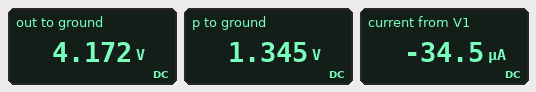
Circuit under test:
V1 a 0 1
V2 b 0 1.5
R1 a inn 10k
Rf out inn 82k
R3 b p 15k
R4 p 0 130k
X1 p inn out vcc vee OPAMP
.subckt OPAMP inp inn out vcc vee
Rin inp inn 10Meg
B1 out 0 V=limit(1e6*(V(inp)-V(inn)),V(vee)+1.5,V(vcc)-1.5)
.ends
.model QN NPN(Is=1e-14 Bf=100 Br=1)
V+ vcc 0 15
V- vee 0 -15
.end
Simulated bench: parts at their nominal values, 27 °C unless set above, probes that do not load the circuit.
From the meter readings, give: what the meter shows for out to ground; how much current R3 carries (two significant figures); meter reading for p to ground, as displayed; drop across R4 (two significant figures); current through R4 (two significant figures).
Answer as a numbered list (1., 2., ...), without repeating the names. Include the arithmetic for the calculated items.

1. 4.172 V
2. (1.5 V - 1.345 V) / 15 kΩ = 10 µA
3. 1.345 V
4. 1.345 V = 1.3 V
5. (1.345 V) / 130 kΩ = 10 µA
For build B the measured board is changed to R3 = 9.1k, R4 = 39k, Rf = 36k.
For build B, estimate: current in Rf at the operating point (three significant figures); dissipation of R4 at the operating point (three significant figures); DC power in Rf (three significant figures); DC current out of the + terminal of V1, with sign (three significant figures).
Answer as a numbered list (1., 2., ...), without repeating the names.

1. 21.6 µA
2. 37.9 µW
3. 16.8 µW
4. -21.6 µA
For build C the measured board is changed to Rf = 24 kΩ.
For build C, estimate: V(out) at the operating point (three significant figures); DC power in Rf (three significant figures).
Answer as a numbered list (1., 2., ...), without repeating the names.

1. 2.17 V
2. 28.5 µW
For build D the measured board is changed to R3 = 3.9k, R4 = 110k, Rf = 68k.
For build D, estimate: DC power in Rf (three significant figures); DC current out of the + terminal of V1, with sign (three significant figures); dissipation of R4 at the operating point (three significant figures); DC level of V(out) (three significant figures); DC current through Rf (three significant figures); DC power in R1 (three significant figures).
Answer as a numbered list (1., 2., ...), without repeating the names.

1. 137 µW
2. -44.9 µA
3. 19.1 µW
4. 4.50 V
5. 44.9 µA
6. 20.1 µW
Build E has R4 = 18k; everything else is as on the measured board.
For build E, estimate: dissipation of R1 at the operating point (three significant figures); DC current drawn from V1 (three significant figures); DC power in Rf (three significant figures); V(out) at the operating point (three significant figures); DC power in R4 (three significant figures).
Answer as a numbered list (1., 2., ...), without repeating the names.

1. 3.31 µW
2. 18.2 µA
3. 27.1 µW
4. -673 mV
5. 37.2 µW
